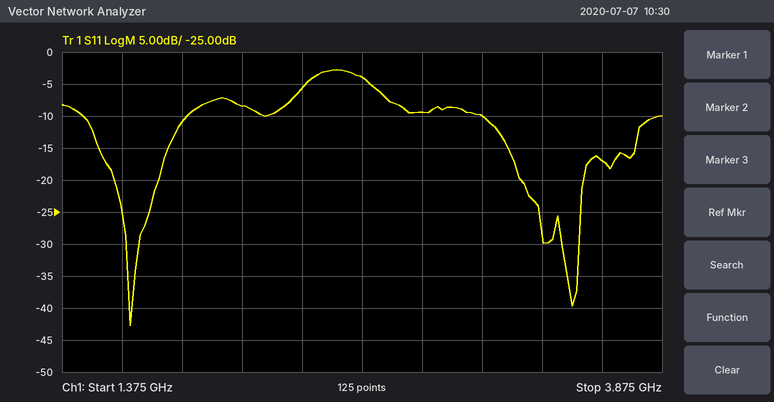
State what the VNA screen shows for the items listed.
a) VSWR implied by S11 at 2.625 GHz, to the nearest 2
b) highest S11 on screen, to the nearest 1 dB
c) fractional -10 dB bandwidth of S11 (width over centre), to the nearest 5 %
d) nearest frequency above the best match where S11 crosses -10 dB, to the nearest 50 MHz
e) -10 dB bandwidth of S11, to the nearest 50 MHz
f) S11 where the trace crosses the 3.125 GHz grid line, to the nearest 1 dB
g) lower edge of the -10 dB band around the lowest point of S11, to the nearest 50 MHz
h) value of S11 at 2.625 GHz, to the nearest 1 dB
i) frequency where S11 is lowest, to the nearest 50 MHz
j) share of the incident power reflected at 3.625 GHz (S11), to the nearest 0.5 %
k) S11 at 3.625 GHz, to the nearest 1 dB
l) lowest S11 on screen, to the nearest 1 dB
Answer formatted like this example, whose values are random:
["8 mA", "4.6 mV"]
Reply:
["4", "-3 dB", "25 %", "1.90 GHz", "450 MHz", "-10 dB", "1.45 GHz", "-4 dB", "1.65 GHz", "2.0 %", "-17 dB", "-43 dB"]
